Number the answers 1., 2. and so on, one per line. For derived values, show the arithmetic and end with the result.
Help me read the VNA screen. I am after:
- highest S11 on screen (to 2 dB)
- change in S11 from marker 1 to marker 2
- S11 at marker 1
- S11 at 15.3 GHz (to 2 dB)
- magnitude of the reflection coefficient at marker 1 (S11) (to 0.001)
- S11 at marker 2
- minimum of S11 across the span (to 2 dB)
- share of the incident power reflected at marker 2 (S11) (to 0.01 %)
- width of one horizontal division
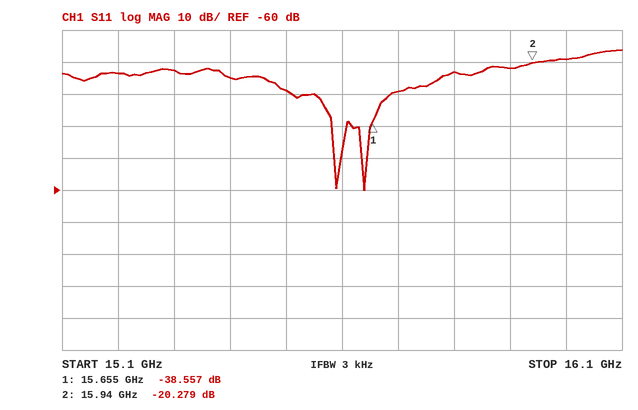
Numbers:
1. -16 dB
2. -20.279 − (-38.557) = 18.278 dB
3. -38.557 dB
4. -22 dB
5. 10^(-38.557/20) ≈ 0.012
6. -20.279 dB
7. -60 dB
8. 10^(-20.279/10) ≈ 0.94 %
9. 100 MHz
